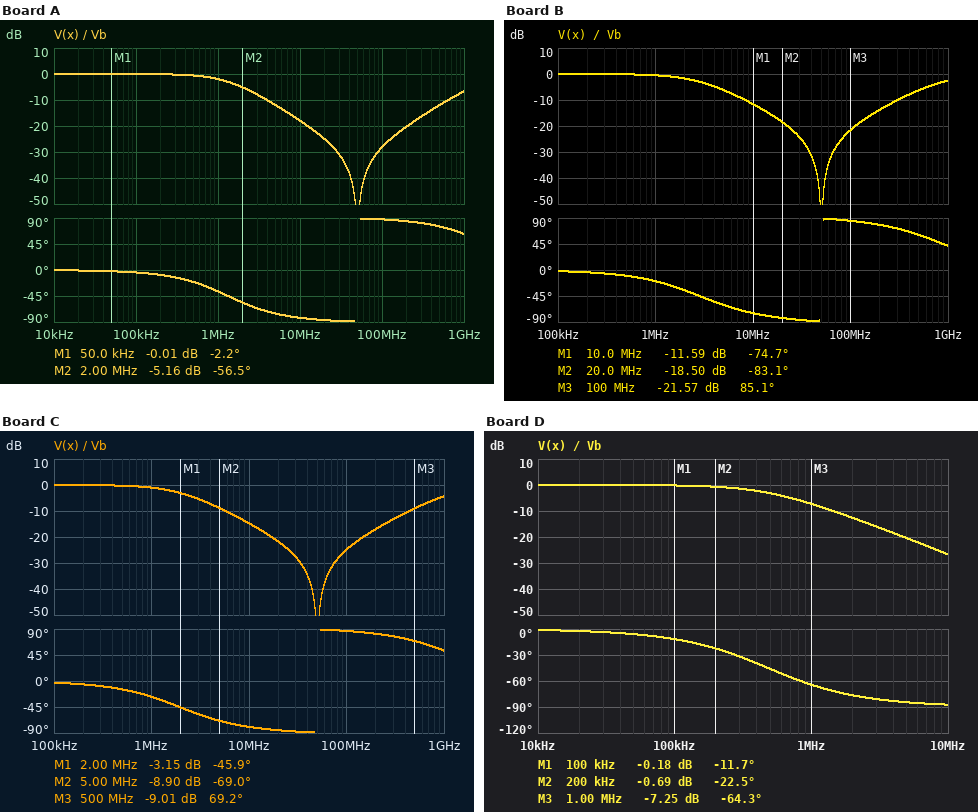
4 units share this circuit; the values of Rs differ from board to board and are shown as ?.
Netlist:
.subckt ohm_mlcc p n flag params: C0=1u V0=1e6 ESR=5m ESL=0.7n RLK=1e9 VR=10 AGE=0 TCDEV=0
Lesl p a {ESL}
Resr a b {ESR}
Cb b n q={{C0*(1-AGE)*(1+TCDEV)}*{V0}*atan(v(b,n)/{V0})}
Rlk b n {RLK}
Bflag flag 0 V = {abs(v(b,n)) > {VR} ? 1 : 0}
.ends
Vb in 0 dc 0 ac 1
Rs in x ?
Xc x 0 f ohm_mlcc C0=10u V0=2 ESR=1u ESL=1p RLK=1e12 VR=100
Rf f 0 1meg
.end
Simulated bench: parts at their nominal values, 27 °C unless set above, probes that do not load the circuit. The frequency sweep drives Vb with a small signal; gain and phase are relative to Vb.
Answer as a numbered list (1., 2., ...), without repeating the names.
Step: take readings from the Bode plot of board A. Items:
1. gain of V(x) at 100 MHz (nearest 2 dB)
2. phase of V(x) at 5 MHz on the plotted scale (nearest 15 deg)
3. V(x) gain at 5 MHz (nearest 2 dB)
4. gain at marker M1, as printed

1. -28 dB
2. -75 deg
3. -12 dB
4. -0.01 dB
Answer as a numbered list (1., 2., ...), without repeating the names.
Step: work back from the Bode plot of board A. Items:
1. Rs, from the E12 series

1. 0.012 Ω
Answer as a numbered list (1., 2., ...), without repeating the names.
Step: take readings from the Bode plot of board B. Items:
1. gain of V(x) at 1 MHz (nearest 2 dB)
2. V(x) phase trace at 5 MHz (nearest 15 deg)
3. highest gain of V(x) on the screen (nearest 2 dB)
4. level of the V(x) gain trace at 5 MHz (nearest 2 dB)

1. 0 dB
2. -60 deg
3. 0 dB
4. -6 dB
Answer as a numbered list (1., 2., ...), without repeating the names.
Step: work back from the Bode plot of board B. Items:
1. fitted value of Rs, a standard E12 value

1. 5.6 mΩ
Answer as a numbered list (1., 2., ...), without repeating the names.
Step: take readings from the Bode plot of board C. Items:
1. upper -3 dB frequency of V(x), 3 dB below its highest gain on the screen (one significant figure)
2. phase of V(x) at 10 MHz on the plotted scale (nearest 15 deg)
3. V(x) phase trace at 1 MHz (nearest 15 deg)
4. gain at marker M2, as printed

1. 2 MHz
2. -75 deg
3. -30 deg
4. -8.90 dB
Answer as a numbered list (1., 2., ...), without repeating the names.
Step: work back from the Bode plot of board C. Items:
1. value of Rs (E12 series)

1. 8.2 mΩ
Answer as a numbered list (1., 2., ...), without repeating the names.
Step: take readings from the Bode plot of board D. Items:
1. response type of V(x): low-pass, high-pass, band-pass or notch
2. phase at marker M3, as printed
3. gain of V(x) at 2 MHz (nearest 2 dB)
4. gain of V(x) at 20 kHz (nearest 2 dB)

1. low-pass
2. -64.3 deg
3. -12 dB
4. 0 dB
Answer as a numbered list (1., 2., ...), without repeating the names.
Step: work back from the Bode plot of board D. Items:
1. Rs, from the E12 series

1. 0.033 Ω
